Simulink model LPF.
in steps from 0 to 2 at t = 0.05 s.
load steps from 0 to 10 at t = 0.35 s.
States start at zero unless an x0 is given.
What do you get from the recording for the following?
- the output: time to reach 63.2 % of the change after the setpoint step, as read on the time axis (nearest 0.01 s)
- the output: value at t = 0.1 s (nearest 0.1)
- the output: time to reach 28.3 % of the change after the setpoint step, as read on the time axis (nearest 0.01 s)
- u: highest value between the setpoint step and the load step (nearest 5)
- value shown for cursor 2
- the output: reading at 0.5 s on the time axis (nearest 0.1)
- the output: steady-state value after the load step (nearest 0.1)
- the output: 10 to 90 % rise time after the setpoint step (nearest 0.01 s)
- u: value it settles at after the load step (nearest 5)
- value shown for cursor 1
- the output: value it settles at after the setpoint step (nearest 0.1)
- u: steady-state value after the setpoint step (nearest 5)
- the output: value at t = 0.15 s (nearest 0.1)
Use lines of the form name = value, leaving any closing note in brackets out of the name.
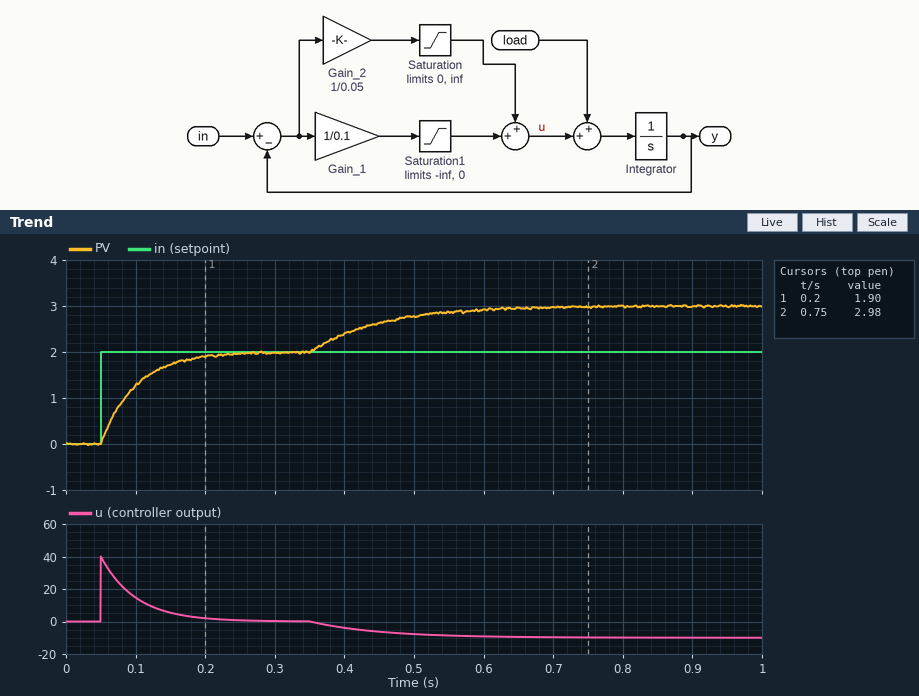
the output: time to reach 63.2 % of the change after the setpoint step, as read on the time axis = 0.10 s
the output: value at t = 0.1 s = 1.3
the output: time to reach 28.3 % of the change after the setpoint step, as read on the time axis = 0.07 s
u: highest value between the setpoint step and the load step = 40
value shown for cursor 2 = 2.98
the output: reading at 0.5 s on the time axis = 2.8
the output: steady-state value after the load step = 3.0
the output: 10 to 90 % rise time after the setpoint step = 0.11 s
u: value it settles at after the load step = -10
value shown for cursor 1 = 1.90
the output: value it settles at after the setpoint step = 2.0
u: steady-state value after the setpoint step = 0
the output: value at t = 0.15 s = 1.7
